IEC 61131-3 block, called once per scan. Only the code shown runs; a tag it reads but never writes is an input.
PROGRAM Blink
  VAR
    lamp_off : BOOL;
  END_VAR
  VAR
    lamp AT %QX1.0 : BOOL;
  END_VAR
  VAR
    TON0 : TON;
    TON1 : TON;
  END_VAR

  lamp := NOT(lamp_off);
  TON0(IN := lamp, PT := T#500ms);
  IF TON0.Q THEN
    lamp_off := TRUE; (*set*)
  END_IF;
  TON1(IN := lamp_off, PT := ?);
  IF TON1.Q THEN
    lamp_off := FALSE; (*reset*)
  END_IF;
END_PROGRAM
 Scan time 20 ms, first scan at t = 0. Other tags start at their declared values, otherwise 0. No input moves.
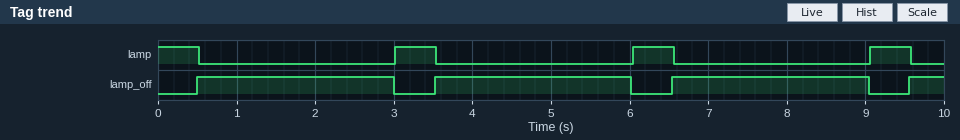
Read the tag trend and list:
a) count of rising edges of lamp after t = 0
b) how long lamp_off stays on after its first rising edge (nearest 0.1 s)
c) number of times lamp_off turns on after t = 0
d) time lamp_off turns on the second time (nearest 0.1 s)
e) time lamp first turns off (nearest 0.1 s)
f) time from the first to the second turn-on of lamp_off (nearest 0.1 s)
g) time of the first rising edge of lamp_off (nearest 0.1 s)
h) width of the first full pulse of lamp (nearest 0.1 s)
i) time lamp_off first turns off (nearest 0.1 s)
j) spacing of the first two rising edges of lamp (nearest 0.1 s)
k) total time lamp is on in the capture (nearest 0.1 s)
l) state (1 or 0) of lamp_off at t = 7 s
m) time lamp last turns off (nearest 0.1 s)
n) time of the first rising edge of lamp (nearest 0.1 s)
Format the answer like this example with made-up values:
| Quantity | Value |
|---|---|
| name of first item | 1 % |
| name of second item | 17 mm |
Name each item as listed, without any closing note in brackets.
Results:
| Quantity | Value |
|---|---|
| count of rising edges of lamp after t = 0 | 3 |
| how long lamp_off stays on after its first rising edge | 2.5 s |
| number of times lamp_off turns on after t = 0 | 4 |
| time lamp_off turns on the second time | 3.5 s |
| time lamp first turns off | 0.5 s |
| time from the first to the second turn-on of lamp_off | 3.0 s |
| time of the first rising edge of lamp_off | 0.5 s |
| width of the first full pulse of lamp | 0.5 s |
| time lamp_off first turns off | 3.0 s |
| spacing of the first two rising edges of lamp | 3.0 s |
| total time lamp is on in the capture | 2.1 s |
| state (1 or 0) of lamp_off at t = 7 s | 1 |
| time lamp last turns off | 9.6 s |
| time of the first rising edge of lamp | 3.0 s |
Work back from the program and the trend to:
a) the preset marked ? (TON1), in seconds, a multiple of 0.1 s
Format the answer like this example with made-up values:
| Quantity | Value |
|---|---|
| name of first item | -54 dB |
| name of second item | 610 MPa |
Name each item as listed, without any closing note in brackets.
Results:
| Quantity | Value |
|---|---|
| the preset marked ? (TON1), in seconds, a multiple of 0.1 s | 2.5 s |
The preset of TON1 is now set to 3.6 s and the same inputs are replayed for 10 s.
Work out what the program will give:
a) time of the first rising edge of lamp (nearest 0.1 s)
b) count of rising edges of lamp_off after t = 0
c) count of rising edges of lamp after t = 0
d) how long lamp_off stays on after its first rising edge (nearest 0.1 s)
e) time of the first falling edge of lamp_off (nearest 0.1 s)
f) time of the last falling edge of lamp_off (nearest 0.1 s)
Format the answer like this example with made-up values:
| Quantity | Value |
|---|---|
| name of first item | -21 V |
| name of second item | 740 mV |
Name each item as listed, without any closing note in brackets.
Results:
| Quantity | Value |
|---|---|
| time of the first rising edge of lamp | 4.1 s |
| count of rising edges of lamp_off after t = 0 | 3 |
| count of rising edges of lamp after t = 0 | 2 |
| how long lamp_off stays on after its first rising edge | 3.6 s |
| time of the first falling edge of lamp_off | 4.1 s |
| time of the last falling edge of lamp_off | 8.2 s |
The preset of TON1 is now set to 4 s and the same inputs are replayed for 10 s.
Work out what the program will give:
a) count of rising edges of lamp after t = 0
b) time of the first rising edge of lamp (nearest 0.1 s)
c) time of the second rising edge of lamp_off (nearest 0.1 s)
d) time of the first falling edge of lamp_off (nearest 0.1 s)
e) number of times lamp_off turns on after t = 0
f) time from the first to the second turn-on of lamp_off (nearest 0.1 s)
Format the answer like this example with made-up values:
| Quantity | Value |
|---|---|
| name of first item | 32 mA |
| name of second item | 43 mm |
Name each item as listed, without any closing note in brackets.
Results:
| Quantity | Value |
|---|---|
| count of rising edges of lamp after t = 0 | 2 |
| time of the first rising edge of lamp | 4.5 s |
| time of the second rising edge of lamp_off | 5.0 s |
| time of the first falling edge of lamp_off | 4.5 s |
| number of times lamp_off turns on after t = 0 | 3 |
| time from the first to the second turn-on of lamp_off | 4.5 s |
